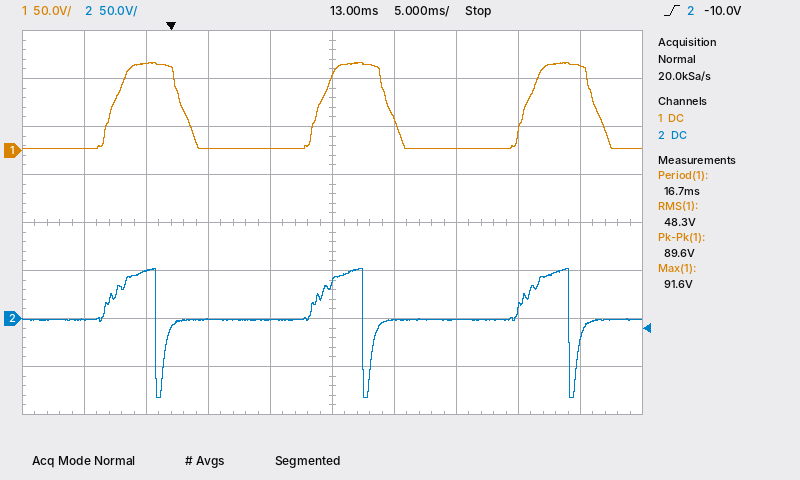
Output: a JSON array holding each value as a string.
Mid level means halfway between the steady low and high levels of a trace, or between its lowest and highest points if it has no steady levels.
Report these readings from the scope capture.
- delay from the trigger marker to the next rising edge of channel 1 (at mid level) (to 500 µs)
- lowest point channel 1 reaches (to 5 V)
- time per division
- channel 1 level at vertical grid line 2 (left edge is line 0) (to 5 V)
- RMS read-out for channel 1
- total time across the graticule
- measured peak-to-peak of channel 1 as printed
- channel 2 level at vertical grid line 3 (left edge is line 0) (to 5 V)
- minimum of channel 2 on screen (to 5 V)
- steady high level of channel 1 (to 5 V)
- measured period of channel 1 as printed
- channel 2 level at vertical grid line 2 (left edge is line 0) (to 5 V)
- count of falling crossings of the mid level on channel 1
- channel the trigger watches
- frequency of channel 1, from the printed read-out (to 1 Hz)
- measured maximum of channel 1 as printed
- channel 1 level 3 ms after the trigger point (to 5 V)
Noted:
["12.0 ms", "0 V", "5 ms", "90 V", "48.3 V", "50 ms", "89.6 V", "0 V", "-80 V", "90 V", "16.7 ms", "50 V", "3", "channel 2", "60 Hz", "91.6 V", "0 V"]
